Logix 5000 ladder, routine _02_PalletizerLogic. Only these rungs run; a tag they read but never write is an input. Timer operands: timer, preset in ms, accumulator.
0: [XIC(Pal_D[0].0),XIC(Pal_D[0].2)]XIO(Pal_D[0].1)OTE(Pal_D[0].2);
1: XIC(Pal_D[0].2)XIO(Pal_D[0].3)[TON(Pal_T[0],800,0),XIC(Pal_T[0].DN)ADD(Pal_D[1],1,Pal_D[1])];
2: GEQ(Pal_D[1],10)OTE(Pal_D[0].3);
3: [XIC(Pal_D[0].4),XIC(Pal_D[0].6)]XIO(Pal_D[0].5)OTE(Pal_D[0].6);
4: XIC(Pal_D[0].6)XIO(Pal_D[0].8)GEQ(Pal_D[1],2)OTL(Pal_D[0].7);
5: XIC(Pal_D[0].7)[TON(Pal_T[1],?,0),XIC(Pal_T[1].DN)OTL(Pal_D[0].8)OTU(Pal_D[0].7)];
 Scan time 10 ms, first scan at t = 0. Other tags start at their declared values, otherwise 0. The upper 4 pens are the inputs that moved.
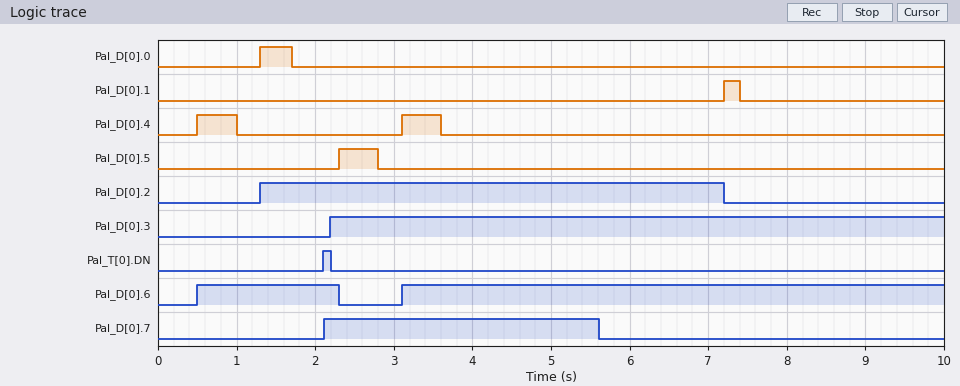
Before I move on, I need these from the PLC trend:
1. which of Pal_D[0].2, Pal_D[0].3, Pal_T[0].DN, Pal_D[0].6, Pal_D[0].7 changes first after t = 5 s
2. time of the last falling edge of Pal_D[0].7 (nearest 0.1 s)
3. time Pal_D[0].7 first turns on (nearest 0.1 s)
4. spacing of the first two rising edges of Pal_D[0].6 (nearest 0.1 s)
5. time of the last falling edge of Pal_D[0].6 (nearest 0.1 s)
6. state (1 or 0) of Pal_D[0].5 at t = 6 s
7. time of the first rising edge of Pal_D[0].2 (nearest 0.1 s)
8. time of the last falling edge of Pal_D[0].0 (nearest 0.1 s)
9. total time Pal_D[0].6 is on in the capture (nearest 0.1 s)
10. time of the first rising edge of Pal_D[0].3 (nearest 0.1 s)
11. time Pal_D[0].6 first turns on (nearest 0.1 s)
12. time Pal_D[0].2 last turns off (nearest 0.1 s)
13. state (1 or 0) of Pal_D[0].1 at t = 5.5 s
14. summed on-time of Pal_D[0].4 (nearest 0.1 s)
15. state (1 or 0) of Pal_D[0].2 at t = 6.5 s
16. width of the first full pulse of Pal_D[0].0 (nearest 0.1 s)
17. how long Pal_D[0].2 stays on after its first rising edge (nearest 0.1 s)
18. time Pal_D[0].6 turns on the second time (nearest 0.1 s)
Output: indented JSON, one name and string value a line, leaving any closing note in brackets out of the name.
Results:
{
  "which of Pal_D[0].2, Pal_D[0].3, Pal_T[0].DN, Pal_D[0].6, Pal_D[0].7 changes first after t = 5 s": "Pal_D[0].7",
  "time of the last falling edge of Pal_D[0].7": "5.6 s",
  "time Pal_D[0].7 first turns on": "2.1 s",
  "spacing of the first two rising edges of Pal_D[0].6": "2.6 s",
  "time of the last falling edge of Pal_D[0].6": "2.3 s",
  "state (1 or 0) of Pal_D[0].5 at t = 6 s": "0",
  "time of the first rising edge of Pal_D[0].2": "1.3 s",
  "time of the last falling edge of Pal_D[0].0": "1.7 s",
  "total time Pal_D[0].6 is on in the capture": "8.7 s",
  "time of the first rising edge of Pal_D[0].3": "2.2 s",
  "time Pal_D[0].6 first turns on": "0.5 s",
  "time Pal_D[0].2 last turns off": "7.2 s",
  "state (1 or 0) of Pal_D[0].1 at t = 5.5 s": "0",
  "summed on-time of Pal_D[0].4": "1.0 s",
  "state (1 or 0) of Pal_D[0].2 at t = 6.5 s": "1",
  "width of the first full pulse of Pal_D[0].0": "0.4 s",
  "how long Pal_D[0].2 stays on after its first rising edge": "5.9 s",
  "time Pal_D[0].6 turns on the second time": "3.1 s"
}
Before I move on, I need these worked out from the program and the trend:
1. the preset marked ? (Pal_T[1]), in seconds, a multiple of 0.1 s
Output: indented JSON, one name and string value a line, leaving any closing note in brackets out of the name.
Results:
{
  "the preset marked ? (Pal_T[1]), in seconds, a multiple of 0.1 s": "3.5 s"
}
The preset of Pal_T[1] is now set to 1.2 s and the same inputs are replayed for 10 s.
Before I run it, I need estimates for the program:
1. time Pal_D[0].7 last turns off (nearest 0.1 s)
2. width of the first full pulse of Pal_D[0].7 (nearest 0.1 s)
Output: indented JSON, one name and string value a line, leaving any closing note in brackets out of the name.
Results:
{
  "time Pal_D[0].7 last turns off": "3.3 s",
  "width of the first full pulse of Pal_D[0].7": "1.2 s"
}
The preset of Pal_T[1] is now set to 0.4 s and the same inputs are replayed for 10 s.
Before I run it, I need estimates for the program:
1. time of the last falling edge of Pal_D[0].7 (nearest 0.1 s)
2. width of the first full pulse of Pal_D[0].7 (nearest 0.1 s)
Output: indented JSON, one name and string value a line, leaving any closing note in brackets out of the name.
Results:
{
  "time of the last falling edge of Pal_D[0].7": "2.5 s",
  "width of the first full pulse of Pal_D[0].7": "0.4 s"
}
